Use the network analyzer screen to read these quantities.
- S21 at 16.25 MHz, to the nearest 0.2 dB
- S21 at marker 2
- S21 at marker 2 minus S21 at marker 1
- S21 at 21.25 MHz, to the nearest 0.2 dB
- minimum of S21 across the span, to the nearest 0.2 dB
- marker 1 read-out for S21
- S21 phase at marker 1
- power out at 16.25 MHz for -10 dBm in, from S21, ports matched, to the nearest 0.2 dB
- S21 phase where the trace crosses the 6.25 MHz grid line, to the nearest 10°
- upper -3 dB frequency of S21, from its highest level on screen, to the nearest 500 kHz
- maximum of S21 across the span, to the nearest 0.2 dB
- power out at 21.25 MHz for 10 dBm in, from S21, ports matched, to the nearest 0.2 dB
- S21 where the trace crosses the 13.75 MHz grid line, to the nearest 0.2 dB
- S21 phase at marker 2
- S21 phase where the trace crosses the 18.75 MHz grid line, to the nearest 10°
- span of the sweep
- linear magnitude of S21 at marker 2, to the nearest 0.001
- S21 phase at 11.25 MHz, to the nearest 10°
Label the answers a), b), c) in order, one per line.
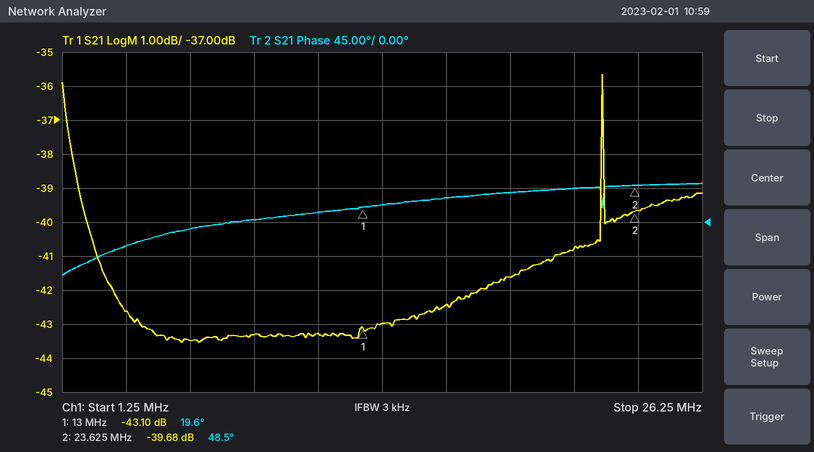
a) -42.4 dB
b) -39.68 dB
c) 3.42 dB
d) -40.8 dB
e) -43.6 dB
f) -43.10 dB
g) 19.6°
h) -52.4 dBm
i) -10°
j) 22.5 MHz
k) -35.6 dB
l) -30.8 dBm
m) -43.0 dB
n) 48.5°
o) 40°
p) 25 MHz
q) 0.010
r) 10°
